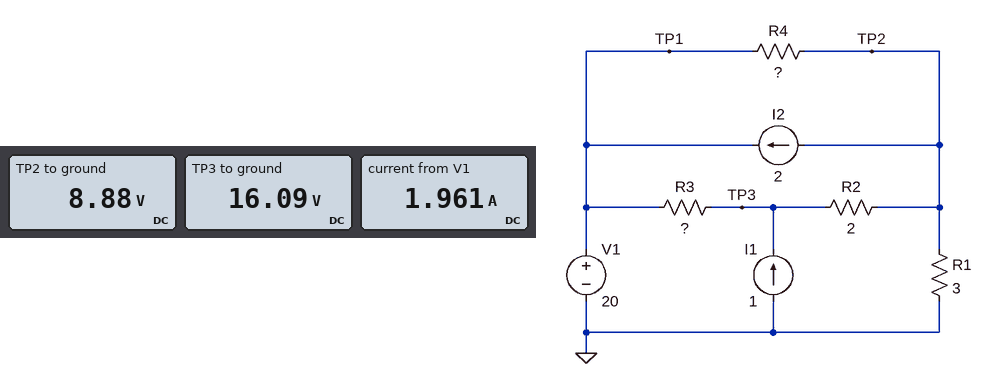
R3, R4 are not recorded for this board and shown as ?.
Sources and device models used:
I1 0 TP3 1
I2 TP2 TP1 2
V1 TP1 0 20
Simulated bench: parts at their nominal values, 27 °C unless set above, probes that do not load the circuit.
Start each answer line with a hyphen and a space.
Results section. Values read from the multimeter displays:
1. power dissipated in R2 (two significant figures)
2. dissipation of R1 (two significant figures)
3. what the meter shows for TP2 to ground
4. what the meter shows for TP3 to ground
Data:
- 26 W
- 26 W
- 8.88 V
- 16.09 V
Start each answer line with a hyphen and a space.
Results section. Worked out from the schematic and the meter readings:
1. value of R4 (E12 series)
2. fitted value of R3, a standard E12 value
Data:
- 8.2 Ω
- 1.5 Ω
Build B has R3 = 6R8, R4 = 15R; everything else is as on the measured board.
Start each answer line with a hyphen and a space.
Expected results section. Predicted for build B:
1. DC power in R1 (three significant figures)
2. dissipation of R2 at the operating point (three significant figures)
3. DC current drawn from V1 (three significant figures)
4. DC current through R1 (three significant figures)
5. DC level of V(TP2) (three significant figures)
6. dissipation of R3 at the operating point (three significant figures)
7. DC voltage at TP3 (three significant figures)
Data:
- 7.15 W
- 12.7 W
- 544 mA
- 1.54 A
- 4.63 V
- 15.7 W
- 9.67 V
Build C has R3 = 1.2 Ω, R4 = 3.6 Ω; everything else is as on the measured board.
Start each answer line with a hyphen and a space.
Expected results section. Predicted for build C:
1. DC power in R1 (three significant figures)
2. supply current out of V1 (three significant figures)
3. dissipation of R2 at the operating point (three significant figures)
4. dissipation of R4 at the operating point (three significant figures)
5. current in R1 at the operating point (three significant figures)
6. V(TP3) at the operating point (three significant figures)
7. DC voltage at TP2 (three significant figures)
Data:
- 40.5 W
- 2.67 A
- 20.2 W
- 22.4 W
- 3.67 A
- 17.4 V
- 11.0 V
